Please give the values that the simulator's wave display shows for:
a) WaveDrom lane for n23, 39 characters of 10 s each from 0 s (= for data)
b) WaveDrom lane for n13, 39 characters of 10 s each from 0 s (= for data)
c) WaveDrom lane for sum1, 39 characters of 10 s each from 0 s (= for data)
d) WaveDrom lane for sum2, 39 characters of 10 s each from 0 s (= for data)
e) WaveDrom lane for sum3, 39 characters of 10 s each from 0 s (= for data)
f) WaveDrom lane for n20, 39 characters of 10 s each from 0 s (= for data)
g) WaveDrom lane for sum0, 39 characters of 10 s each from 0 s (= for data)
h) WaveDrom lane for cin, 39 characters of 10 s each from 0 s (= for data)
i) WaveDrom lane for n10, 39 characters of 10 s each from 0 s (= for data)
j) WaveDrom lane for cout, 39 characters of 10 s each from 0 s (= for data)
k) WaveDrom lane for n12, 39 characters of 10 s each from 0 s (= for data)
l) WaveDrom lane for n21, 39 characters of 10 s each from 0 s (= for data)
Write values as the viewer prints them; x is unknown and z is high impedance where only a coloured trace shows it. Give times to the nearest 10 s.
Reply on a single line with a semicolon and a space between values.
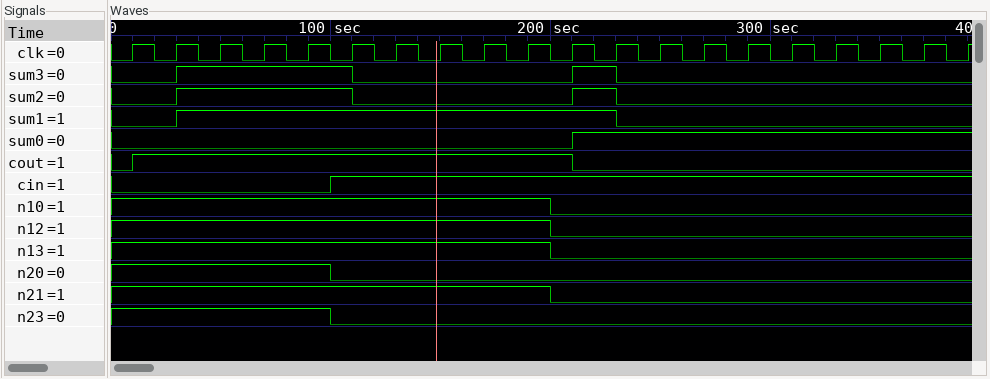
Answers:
{name: 'n23', wave: '1.........0............................'}; {name: 'n13', wave: '1...................0..................'}; {name: 'sum1', wave: '0..1...................0...............'}; {name: 'sum2', wave: '0..1.......0.........1.0...............'}; {name: 'sum3', wave: '0..1.......0.........1.0...............'}; {name: 'n20', wave: '1.........0............................'}; {name: 'sum0', wave: '0....................1.................'}; {name: 'cin', wave: '0.........1............................'}; {name: 'n10', wave: '1...................0..................'}; {name: 'cout', wave: '01...................0.................'}; {name: 'n12', wave: '1...................0..................'}; {name: 'n21', wave: '1...................0..................'}
